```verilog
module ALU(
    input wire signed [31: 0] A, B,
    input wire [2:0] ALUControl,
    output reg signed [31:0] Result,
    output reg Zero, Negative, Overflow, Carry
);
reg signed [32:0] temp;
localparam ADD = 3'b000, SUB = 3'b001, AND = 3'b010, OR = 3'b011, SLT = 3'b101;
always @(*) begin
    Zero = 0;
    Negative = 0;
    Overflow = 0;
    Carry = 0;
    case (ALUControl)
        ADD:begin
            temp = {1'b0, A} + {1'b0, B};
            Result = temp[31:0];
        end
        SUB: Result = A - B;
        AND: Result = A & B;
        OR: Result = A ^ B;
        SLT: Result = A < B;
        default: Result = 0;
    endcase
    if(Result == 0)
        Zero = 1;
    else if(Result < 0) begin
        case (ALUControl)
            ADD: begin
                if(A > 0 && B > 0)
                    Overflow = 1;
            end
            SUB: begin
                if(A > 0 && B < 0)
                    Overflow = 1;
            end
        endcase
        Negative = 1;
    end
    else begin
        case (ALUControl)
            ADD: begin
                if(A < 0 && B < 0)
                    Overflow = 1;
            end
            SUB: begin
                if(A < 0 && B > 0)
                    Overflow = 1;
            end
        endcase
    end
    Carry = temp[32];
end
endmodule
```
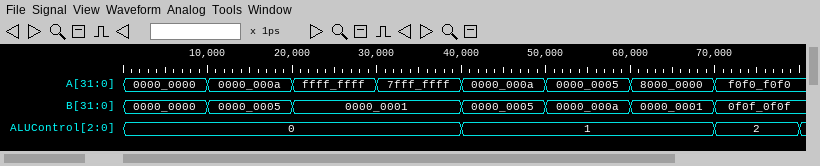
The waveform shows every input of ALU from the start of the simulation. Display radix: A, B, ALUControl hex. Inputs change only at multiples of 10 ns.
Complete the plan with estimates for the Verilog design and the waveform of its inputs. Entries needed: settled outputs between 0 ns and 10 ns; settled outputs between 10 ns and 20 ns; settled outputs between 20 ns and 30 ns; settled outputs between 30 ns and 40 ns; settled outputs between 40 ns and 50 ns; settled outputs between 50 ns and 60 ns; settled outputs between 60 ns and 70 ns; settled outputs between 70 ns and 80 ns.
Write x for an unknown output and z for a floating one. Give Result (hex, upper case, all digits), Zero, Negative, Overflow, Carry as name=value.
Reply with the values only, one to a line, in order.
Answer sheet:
Result=00000000, Zero=1, Negative=0, Overflow=0, Carry=0
Result=0000000F, Zero=0, Negative=0, Overflow=0, Carry=0
Result=00000000, Zero=1, Negative=0, Overflow=0, Carry=1
Result=80000000, Zero=0, Negative=1, Overflow=1, Carry=0
Result=00000005, Zero=0, Negative=0, Overflow=0, Carry=0
Result=FFFFFFFB, Zero=0, Negative=1, Overflow=0, Carry=0
Result=7FFFFFFF, Zero=0, Negative=0, Overflow=1, Carry=0
Result=00000000, Zero=1, Negative=0, Overflow=0, Carry=0
